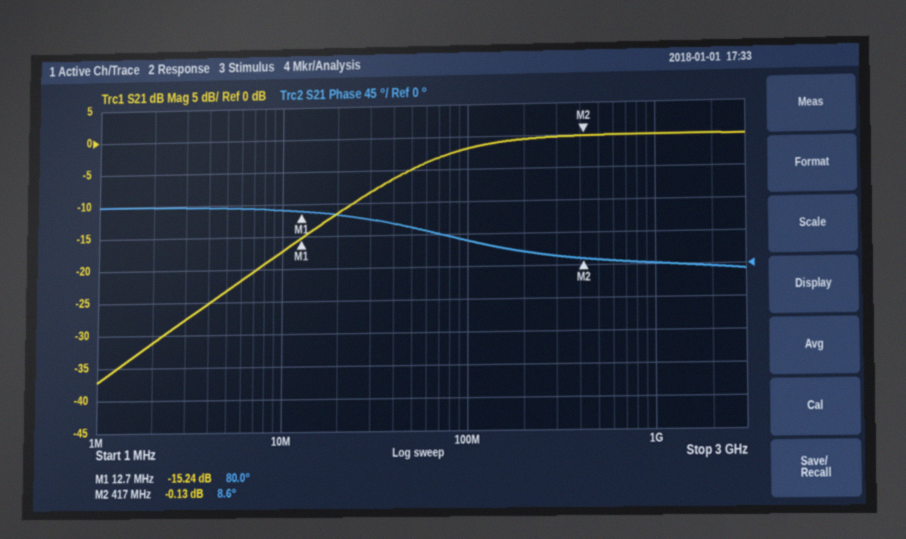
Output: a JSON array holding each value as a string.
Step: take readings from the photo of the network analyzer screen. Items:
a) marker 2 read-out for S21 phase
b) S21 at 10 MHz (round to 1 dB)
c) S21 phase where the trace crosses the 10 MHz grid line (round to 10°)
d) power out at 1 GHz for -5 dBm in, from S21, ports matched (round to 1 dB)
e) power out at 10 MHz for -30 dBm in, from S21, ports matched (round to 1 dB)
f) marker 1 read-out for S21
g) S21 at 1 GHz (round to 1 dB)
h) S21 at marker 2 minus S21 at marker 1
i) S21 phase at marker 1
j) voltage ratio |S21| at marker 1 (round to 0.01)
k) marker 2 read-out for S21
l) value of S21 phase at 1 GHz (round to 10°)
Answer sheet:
["8.6°", "-17 dB", "80°", "-5 dBm", "-47 dBm", "-15.24 dB", "0 dB", "15.11 dB", "80.0°", "0.17", "-0.13 dB", "0°"]
